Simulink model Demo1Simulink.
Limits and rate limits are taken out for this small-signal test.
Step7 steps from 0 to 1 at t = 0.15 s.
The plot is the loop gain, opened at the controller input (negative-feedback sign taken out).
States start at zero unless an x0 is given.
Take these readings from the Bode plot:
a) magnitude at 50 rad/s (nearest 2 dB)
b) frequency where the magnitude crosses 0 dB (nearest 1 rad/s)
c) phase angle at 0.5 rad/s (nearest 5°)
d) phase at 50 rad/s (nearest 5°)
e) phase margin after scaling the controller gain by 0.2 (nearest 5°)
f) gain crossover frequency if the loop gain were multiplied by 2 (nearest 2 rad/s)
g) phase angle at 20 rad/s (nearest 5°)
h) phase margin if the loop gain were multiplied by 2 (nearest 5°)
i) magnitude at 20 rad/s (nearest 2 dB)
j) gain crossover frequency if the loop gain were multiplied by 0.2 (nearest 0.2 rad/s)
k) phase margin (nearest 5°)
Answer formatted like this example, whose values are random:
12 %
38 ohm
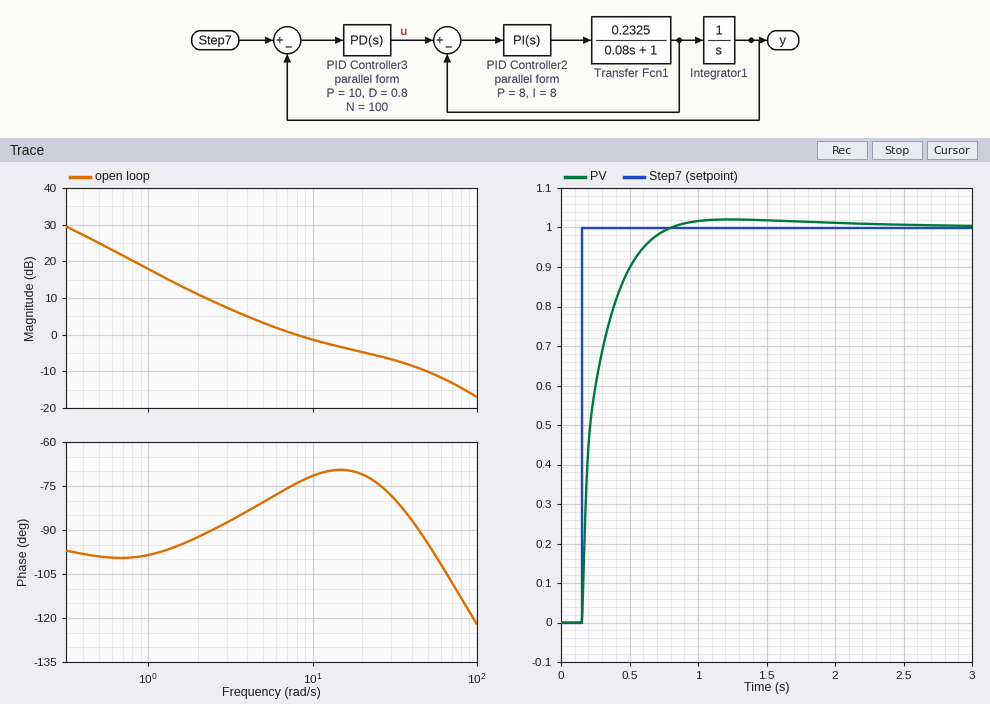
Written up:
-10 dB
8 rad/s
-100°
-95°
85°
26 rad/s
-70°
105°
-4 dB
1.4 rad/s
105°
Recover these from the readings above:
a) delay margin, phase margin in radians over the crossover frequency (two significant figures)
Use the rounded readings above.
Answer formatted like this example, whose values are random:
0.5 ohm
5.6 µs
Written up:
0.23 s
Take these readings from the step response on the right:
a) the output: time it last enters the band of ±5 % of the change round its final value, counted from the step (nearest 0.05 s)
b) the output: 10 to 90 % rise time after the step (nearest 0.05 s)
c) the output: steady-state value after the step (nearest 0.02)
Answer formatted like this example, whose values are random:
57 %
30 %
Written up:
0.45 s
0.35 s
1.00
